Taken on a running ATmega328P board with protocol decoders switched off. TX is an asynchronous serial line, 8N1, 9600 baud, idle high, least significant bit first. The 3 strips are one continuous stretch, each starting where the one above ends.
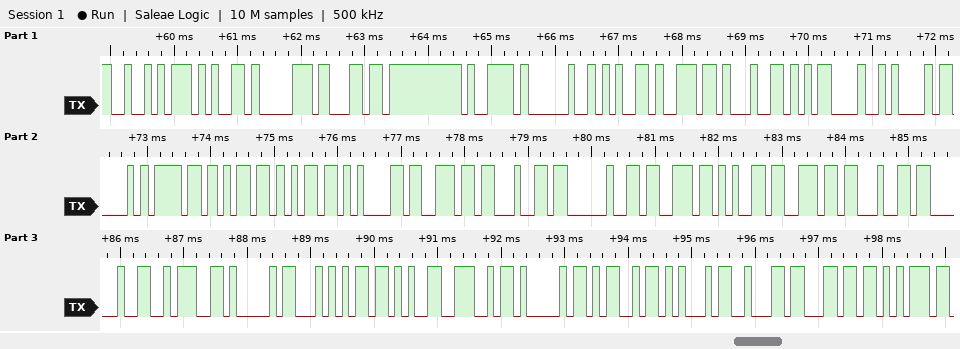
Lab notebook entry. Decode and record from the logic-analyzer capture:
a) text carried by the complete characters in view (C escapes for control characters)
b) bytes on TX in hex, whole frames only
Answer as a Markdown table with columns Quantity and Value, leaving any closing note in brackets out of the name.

| Quantity | Value |
|---|---|
| text carried by the complete characters in view | "Reply end\r\nCommand send :AT+NAMEblu" |
| bytes on TX in hex, whole frames only | 0x52 0x65 0x70 0x6C 0x79 0x20 0x65 0x6E 0x64 0x0D 0x0A 0x43 0x6F 0x6D 0x6D 0x61 0x6E 0x64 0x20 0x73 0x65 0x6E 0x64 0x20 0x3A 0x41 0x54 0x2B 0x4E 0x41 0x4D 0x45 0x62 0x6C 0x75 |
